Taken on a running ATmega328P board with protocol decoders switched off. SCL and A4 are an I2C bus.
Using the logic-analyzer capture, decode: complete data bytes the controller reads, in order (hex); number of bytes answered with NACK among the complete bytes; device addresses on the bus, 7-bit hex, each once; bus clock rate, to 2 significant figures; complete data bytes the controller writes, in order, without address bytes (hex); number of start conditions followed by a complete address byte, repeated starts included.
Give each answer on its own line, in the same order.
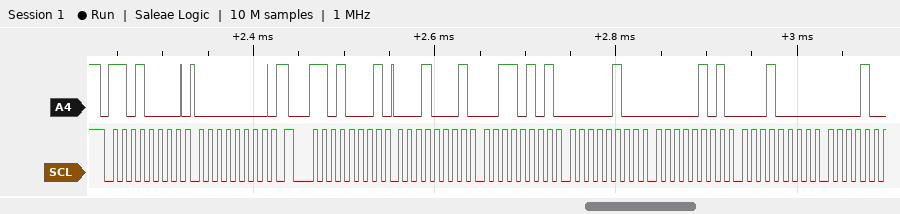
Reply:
11 35 04 05 10
0
0x68
100 kHz
00
2
